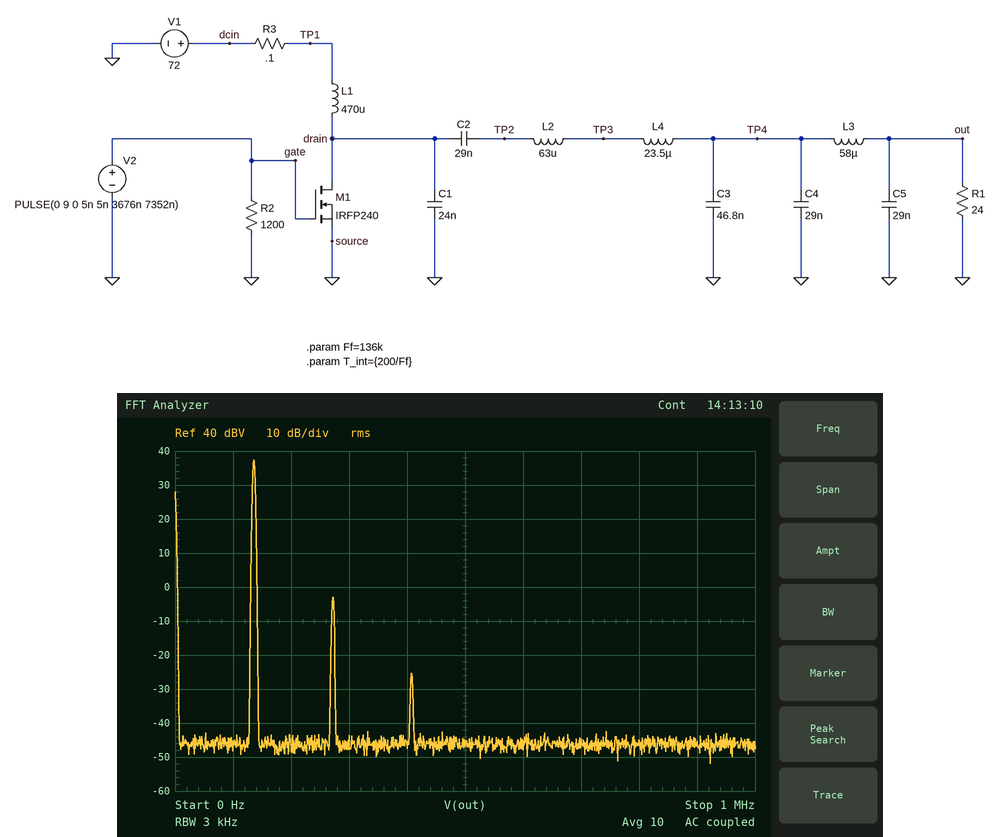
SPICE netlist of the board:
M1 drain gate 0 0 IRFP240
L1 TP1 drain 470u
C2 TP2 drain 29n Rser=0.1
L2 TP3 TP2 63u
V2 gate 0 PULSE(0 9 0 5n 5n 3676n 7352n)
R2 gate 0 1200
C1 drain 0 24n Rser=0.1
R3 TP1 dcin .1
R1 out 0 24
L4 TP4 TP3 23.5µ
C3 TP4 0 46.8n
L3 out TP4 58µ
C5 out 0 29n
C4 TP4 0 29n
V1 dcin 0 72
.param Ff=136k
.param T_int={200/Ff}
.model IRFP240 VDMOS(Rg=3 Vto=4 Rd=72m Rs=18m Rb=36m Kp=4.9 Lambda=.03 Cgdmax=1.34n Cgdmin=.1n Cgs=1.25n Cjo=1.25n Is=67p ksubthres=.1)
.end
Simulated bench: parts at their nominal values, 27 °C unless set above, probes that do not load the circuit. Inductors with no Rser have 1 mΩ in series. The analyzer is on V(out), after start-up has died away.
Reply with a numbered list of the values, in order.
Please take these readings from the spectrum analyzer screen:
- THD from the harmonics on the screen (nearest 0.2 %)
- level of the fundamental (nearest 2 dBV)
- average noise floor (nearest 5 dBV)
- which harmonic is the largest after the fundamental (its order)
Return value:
1. 1.0 %
2. 38 dBV
3. -45 dBV
4. 2
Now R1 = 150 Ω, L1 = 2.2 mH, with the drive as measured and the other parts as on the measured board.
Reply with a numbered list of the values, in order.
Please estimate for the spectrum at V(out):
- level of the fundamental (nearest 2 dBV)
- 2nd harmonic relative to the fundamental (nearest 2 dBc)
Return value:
1. 42 dBV
2. -50 dBc
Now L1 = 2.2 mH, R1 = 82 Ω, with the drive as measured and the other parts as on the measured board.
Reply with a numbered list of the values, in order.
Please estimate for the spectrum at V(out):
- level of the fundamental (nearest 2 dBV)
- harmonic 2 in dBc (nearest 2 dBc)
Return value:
1. 42 dBV
2. -48 dBc
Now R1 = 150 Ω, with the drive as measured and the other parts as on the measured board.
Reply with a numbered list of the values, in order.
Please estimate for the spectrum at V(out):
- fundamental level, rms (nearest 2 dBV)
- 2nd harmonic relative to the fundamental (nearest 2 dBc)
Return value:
1. 42 dBV
2. -50 dBc
